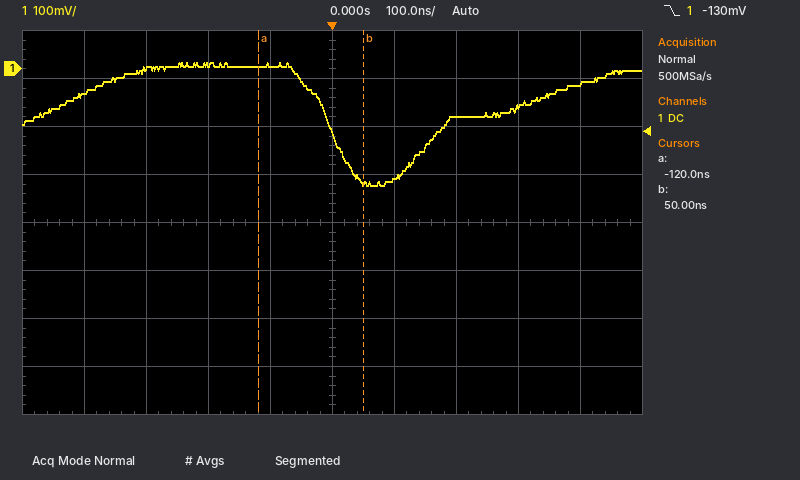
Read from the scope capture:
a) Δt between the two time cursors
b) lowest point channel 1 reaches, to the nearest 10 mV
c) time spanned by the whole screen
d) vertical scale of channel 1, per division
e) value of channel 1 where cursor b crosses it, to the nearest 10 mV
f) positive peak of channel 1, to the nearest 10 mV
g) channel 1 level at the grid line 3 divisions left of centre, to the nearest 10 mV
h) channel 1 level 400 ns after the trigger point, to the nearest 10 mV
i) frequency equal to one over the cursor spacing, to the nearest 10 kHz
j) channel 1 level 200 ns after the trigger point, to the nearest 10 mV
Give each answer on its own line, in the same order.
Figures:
170 ns
-240 mV
1 µs
100 mV
-240 mV
10 mV
0 mV
-30 mV
5.88 MHz
-100 mV
